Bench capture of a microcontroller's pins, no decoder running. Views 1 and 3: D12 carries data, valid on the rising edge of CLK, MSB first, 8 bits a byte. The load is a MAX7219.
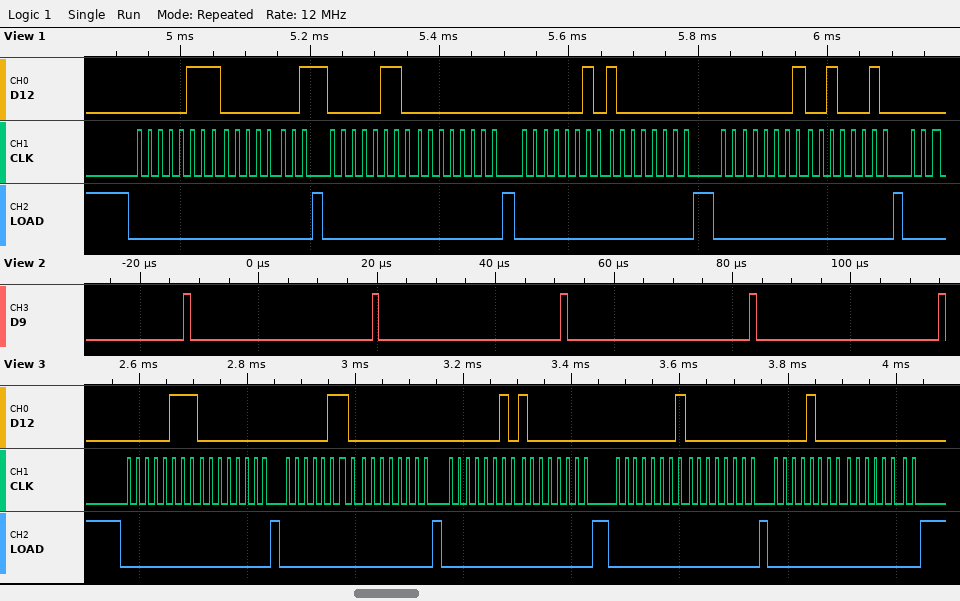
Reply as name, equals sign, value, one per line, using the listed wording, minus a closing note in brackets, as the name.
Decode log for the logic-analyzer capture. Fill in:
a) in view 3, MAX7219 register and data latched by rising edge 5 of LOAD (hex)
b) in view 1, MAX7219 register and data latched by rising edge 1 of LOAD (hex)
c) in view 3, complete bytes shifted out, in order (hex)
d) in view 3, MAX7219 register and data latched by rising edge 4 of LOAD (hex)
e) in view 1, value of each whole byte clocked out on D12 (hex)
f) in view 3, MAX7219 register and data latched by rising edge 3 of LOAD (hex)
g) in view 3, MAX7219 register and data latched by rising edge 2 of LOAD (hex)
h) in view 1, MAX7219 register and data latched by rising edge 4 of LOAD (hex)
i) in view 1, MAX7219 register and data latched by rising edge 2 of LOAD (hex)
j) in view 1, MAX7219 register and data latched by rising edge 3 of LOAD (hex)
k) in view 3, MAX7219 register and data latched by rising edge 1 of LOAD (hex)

in view 3, MAX7219 register and data latched by rising edge 5 of LOAD = register 0x8, data 0x00
in view 1, MAX7219 register and data latched by rising edge 1 of LOAD = register 0x7, data 0x01
in view 3, complete bytes shifted out, in order = 07 00 06 00 02 80 01 00 08 00
in view 3, MAX7219 register and data latched by rising edge 4 of LOAD = register 0x1, data 0x00
in view 1, value of each whole byte clocked out on D12 = 07 01 06 00 02 80 01 22
in view 3, MAX7219 register and data latched by rising edge 3 of LOAD = register 0x2, data 0x80
in view 3, MAX7219 register and data latched by rising edge 2 of LOAD = register 0x6, data 0x00
in view 1, MAX7219 register and data latched by rising edge 4 of LOAD = register 0x1, data 0x22
in view 1, MAX7219 register and data latched by rising edge 2 of LOAD = register 0x6, data 0x00
in view 1, MAX7219 register and data latched by rising edge 3 of LOAD = register 0x2, data 0x80
in view 3, MAX7219 register and data latched by rising edge 1 of LOAD = register 0x7, data 0x00
